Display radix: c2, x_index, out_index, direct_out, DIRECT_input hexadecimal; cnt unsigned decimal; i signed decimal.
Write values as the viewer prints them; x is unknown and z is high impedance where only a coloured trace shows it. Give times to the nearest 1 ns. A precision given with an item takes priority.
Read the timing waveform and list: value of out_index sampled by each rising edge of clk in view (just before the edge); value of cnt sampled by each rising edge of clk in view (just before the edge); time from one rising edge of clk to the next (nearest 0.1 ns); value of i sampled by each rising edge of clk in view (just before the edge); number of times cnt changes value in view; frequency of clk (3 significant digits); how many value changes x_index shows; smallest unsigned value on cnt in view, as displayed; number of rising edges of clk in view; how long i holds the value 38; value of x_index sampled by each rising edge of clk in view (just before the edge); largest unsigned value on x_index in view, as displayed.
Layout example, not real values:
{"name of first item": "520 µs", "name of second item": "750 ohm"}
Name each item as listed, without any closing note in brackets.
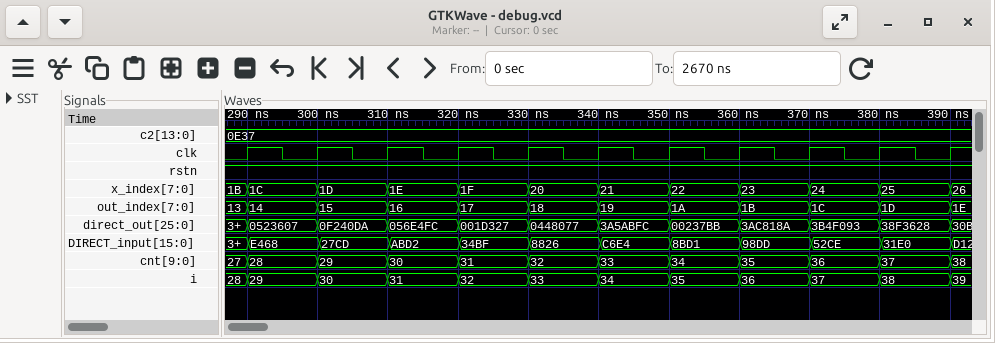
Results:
{"value of out_index sampled by each rising edge of clk in view": "13, 14, 15, 16, 17, 18, 19, 1A, 1B, 1C, 1D", "value of cnt sampled by each rising edge of clk in view": "27, 28, 29, 30, 31, 32, 33, 34, 35, 36, 37", "time from one rising edge of clk to the next": "10 ns", "value of i sampled by each rising edge of clk in view": "28, 29, 30, 31, 32, 33, 34, 35, 36, 37, 38", "number of times cnt changes value in view": "11", "frequency of clk": "100 MHz", "how many value changes x_index shows": "11", "smallest unsigned value on cnt in view, as displayed": "27", "number of rising edges of clk in view": "11", "how long i holds the value 38": "10 ns", "value of x_index sampled by each rising edge of clk in view": "1B, 1C, 1D, 1E, 1F, 20, 21, 22, 23, 24, 25", "largest unsigned value on x_index in view, as displayed": "26"}
